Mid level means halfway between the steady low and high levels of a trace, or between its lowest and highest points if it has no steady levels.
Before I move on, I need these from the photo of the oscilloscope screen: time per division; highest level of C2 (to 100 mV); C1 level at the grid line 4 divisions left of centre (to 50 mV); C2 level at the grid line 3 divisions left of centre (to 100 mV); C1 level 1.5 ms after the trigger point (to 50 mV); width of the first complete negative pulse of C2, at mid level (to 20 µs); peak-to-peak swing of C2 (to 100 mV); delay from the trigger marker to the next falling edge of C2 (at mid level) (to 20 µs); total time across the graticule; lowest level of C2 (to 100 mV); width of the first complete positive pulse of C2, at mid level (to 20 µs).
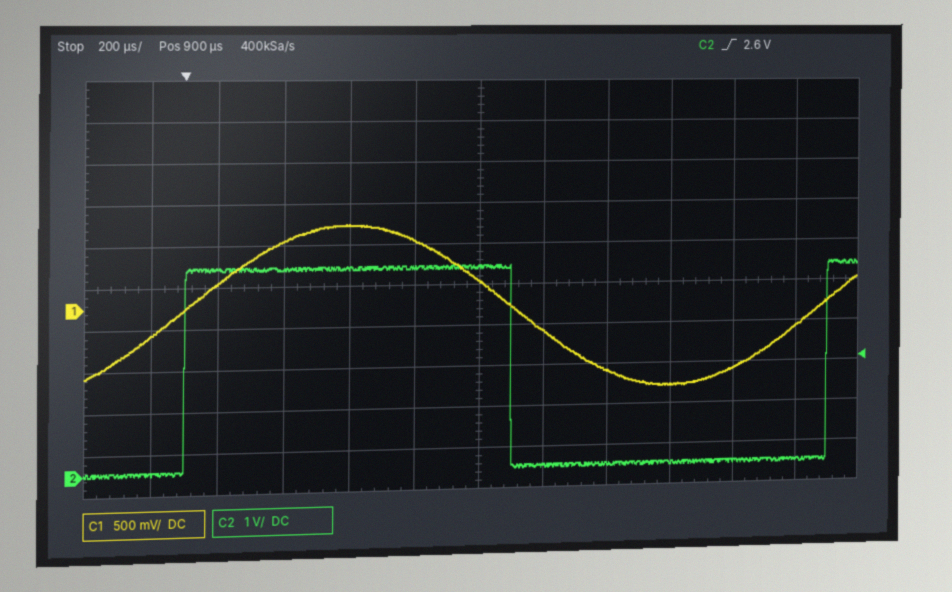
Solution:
200 µs
5.0 V
300 mV
4.9 V
-1.00 V
1.00 ms
5.0 V
1.00 ms
2.4 ms
0.0 V
1.00 ms
